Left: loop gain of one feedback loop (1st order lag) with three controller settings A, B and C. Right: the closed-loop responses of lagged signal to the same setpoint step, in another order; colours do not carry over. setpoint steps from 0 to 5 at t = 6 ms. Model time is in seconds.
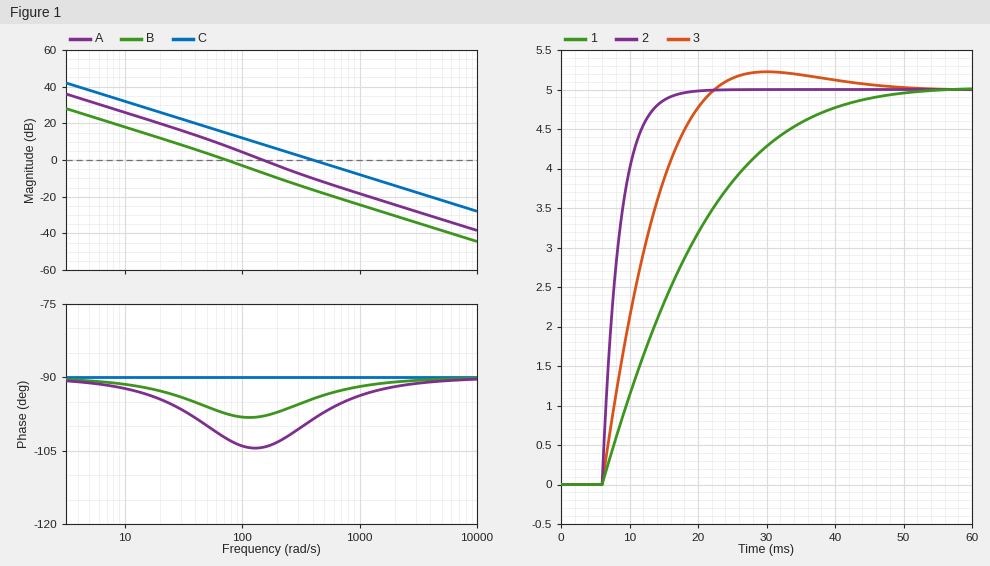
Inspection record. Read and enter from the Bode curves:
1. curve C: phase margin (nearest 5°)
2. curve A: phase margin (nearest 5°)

90°
75°
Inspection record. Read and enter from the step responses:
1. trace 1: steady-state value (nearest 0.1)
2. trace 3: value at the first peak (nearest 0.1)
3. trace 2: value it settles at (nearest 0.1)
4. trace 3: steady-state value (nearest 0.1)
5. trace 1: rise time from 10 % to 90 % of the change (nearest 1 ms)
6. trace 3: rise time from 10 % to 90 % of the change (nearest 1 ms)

5.0
5.2
5.0
5.0
26 ms
11 ms
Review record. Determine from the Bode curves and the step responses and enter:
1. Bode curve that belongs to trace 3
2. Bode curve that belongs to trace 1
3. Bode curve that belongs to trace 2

A
B
C
